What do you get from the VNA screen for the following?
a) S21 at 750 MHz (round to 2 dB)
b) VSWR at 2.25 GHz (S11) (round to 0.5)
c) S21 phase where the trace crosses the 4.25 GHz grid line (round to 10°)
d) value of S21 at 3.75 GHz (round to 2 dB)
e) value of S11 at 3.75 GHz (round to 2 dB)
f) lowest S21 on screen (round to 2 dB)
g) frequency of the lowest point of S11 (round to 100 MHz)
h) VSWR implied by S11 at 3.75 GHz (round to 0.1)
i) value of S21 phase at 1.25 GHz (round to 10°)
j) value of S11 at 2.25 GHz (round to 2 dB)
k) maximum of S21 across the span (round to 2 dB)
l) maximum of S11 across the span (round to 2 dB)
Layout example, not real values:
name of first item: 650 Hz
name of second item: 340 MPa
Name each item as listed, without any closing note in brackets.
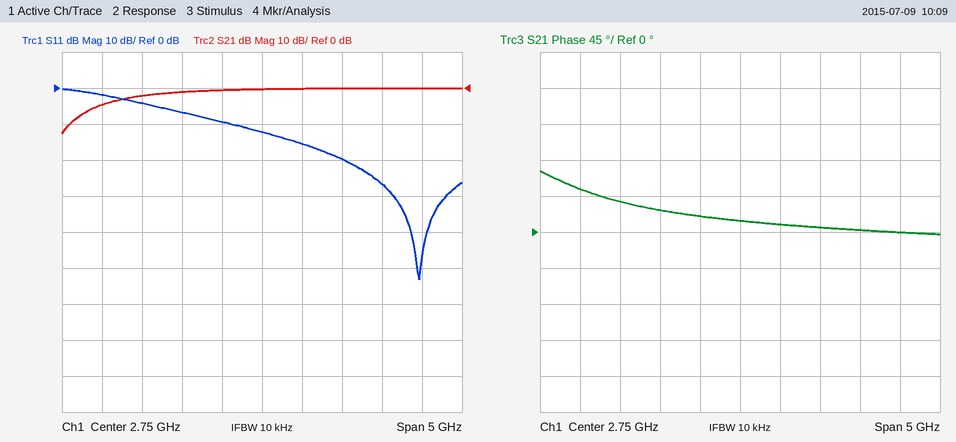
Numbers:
S21 at 750 MHz: -4 dB
VSWR at 2.25 GHz (S11): 2.0
S21 phase where the trace crosses the 4.25 GHz grid line: 0°
value of S21 at 3.75 GHz: 0 dB
value of S11 at 3.75 GHz: -20 dB
lowest S21 on screen: -12 dB
frequency of the lowest point of S11: 4.7 GHz
VSWR implied by S11 at 3.75 GHz: 1.2
value of S21 phase at 1.25 GHz: 40°
value of S11 at 2.25 GHz: -10 dB
maximum of S21 across the span: 0 dB
maximum of S11 across the span: 0 dB
